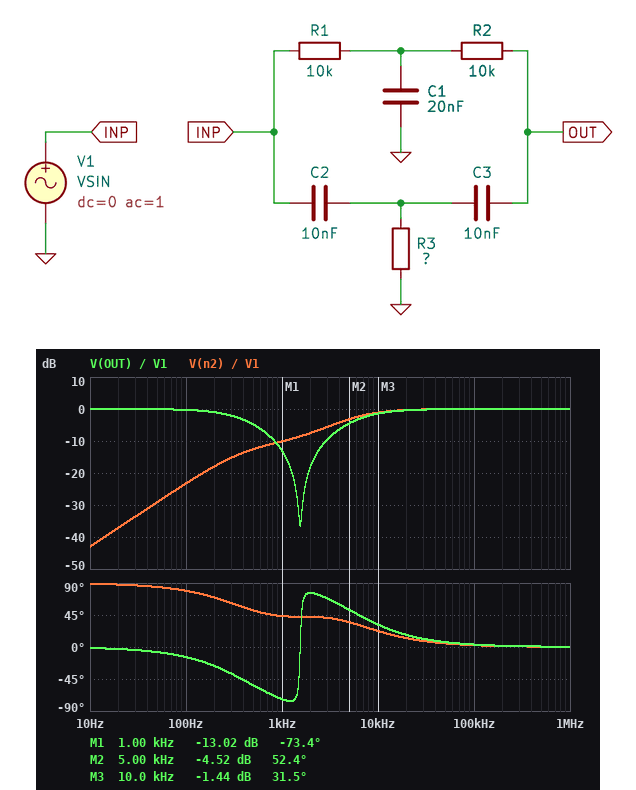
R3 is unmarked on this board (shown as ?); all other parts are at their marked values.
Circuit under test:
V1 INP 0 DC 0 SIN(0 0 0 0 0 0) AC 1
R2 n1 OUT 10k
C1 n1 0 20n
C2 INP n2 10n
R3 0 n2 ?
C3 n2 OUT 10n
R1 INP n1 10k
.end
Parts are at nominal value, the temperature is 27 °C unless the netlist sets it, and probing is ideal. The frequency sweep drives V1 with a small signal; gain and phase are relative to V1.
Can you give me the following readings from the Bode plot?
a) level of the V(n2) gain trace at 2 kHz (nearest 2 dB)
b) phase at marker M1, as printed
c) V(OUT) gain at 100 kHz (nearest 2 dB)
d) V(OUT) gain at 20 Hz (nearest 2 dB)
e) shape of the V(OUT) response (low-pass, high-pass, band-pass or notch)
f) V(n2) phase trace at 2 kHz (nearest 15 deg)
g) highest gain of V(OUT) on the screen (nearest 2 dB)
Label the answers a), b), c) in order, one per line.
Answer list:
a) -8 dB
b) -73.4 deg
c) 0 dB
d) 0 dB
e) notch
f) 45 deg
g) 0 dB
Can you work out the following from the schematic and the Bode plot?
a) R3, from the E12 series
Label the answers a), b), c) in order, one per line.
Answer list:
a) 5.6 kΩ
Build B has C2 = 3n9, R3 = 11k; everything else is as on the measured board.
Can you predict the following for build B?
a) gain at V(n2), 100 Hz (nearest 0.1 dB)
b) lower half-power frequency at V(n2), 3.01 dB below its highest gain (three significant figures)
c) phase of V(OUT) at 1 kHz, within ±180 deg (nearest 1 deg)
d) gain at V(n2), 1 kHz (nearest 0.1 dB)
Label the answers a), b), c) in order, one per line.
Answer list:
a) -20.7 dB
b) 9.33 kHz
c) -64 deg
d) -10.9 dB
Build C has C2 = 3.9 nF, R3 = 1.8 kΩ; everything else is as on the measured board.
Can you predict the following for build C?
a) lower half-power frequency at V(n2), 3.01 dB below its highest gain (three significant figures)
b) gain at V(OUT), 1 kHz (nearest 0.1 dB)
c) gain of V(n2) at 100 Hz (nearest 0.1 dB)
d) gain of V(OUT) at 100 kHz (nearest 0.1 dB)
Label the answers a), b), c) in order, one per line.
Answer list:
a) 27.3 kHz
b) -8.8 dB
c) -36.3 dB
d) -0.3 dB
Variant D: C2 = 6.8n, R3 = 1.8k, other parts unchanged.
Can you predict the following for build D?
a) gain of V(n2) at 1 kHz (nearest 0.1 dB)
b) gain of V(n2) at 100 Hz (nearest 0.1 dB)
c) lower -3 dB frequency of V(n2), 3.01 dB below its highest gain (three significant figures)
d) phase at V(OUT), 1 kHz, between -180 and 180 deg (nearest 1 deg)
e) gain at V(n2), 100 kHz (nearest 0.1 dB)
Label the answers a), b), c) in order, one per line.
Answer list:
a) -21.1 dB
b) -34.6 dB
c) 15.9 kHz
d) -85 deg
e) -0.1 dB
